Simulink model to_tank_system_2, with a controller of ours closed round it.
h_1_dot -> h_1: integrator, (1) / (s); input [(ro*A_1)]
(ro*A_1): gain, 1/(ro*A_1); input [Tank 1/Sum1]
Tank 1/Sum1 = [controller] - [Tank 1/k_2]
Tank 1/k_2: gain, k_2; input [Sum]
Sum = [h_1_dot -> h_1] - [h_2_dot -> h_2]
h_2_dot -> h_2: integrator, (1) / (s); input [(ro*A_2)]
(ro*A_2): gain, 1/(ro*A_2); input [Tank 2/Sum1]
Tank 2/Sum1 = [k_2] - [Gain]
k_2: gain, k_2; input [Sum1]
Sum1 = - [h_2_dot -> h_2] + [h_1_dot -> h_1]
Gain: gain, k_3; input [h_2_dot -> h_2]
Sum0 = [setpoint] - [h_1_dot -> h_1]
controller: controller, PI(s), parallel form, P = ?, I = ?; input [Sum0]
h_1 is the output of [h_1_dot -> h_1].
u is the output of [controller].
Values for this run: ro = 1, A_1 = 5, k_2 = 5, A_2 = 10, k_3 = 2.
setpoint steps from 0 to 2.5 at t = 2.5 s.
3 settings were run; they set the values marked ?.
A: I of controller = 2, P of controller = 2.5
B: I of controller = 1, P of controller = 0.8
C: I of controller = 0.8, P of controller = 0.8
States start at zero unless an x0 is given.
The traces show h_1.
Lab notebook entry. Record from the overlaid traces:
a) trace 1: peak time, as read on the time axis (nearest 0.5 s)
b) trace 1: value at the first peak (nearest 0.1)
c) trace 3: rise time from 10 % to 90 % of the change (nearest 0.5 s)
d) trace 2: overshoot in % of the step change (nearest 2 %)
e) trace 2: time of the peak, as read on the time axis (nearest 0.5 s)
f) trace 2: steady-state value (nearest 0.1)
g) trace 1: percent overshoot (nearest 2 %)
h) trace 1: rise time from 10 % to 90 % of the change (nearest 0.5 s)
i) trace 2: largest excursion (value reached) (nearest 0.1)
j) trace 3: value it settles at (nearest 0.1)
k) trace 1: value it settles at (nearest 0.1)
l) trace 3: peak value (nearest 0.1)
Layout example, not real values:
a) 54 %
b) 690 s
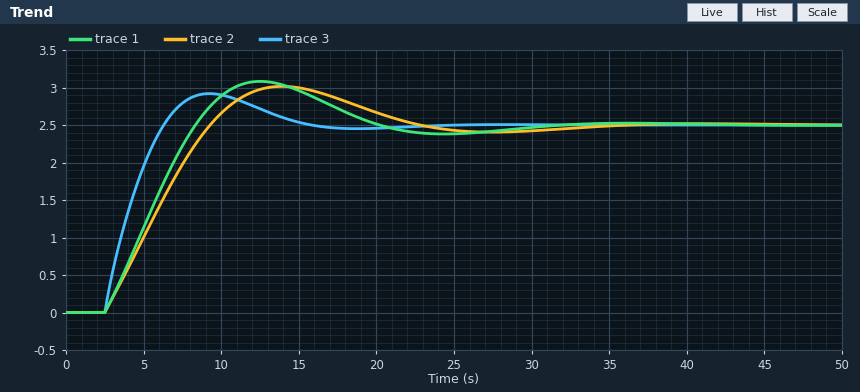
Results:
a) 12.5 s
b) 3.1
c) 3.0 s
d) 20 %
e) 14.0 s
f) 2.5
g) 24 %
h) 4.5 s
i) 3.0
j) 2.5
k) 2.5
l) 2.9
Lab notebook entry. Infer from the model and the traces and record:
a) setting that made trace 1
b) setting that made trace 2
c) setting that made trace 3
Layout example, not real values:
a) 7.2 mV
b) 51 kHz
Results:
a) B
b) C
c) A
